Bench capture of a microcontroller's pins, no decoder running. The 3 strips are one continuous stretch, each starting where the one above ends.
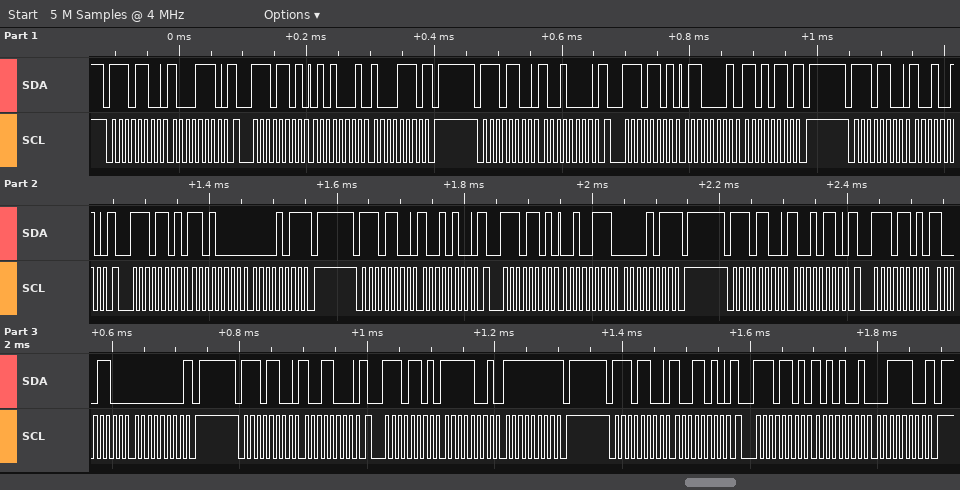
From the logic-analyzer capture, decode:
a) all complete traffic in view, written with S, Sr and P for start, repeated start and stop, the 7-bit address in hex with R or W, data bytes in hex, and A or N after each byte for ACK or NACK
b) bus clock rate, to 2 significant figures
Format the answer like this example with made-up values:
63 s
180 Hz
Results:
S 76W A 8E A Sr 76R A 51 A 8E N P S 76W A 90 A Sr 76R A 61 A D6 N P S 76W A 92 A Sr 76R A D0 A 0B N P S 76W A 94 A Sr 76R A 27 A 0B N P S 76W A 96 A Sr 76R A 8C A 00 N P S 76W A 98 A Sr 76R A F9 A FF N P S 76W A 9A A Sr 76R A A9 A 3C N P
100 kHz
